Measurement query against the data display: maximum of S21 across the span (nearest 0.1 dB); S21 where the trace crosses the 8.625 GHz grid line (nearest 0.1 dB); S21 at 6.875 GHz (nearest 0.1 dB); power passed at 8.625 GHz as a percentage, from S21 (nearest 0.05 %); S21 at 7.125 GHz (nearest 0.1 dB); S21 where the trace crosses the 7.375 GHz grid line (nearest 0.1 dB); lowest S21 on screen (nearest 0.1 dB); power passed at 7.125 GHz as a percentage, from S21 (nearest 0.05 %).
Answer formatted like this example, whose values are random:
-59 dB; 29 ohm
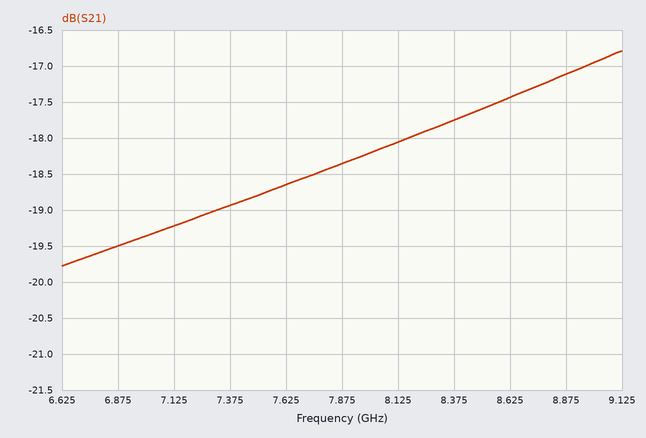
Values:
-16.8 dB; -17.4 dB; -19.5 dB; 1.80 %; -19.2 dB; -18.9 dB; -19.8 dB; 1.20 %
